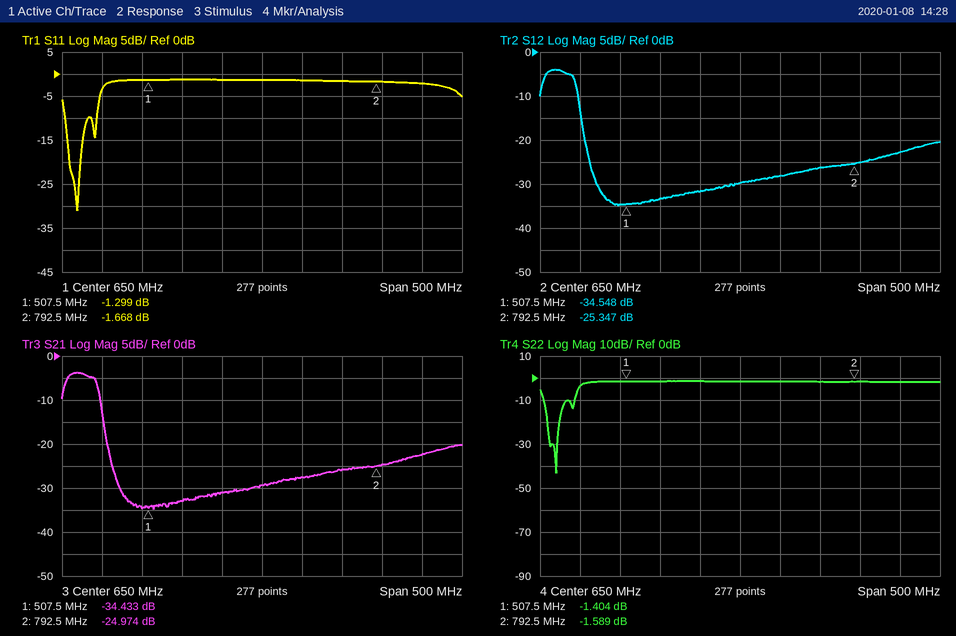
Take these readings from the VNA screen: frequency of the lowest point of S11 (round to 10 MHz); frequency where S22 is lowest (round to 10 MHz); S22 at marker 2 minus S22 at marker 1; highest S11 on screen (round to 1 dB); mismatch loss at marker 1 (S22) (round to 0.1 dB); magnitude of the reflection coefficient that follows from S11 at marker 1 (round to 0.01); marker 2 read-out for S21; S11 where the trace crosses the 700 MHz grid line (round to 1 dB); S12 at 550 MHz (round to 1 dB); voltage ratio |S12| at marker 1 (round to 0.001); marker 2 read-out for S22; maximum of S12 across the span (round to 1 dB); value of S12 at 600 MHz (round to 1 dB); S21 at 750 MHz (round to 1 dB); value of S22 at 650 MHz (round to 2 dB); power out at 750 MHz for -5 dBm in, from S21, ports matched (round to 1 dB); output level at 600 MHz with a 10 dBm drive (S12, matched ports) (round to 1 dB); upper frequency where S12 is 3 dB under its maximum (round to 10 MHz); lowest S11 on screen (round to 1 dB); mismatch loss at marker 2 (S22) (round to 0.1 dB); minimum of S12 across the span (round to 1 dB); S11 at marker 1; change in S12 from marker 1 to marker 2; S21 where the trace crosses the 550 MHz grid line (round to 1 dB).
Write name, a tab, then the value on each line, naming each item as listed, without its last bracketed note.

frequency of the lowest point of S11	420 MHz
frequency where S22 is lowest	420 MHz
S22 at marker 2 minus S22 at marker 1	-0.185 dB
highest S11 on screen	-1 dB
mismatch loss at marker 1 (S22)	5.6 dB
magnitude of the reflection coefficient that follows from S11 at marker 1	0.86
marker 2 read-out for S21	-24.974 dB
S11 where the trace crosses the 700 MHz grid line	-1 dB
S12 at 550 MHz	-33 dB
voltage ratio |S12| at marker 1	0.019
marker 2 read-out for S22	-1.589 dB
maximum of S12 across the span	-4 dB
value of S12 at 600 MHz	-32 dB
S21 at 750 MHz	-26 dB
value of S22 at 650 MHz	-2 dB
power out at 750 MHz for -5 dBm in, from S21, ports matched	-31 dBm
output level at 600 MHz with a 10 dBm drive (S12, matched ports)	-22 dBm
upper frequency where S12 is 3 dB under its maximum	440 MHz
lowest S11 on screen	-31 dB
mismatch loss at marker 2 (S22)	5.1 dB
minimum of S12 across the span	-35 dB
S11 at marker 1	-1.299 dB
change in S12 from marker 1 to marker 2	9.201 dB
S21 where the trace crosses the 550 MHz grid line	-33 dB
